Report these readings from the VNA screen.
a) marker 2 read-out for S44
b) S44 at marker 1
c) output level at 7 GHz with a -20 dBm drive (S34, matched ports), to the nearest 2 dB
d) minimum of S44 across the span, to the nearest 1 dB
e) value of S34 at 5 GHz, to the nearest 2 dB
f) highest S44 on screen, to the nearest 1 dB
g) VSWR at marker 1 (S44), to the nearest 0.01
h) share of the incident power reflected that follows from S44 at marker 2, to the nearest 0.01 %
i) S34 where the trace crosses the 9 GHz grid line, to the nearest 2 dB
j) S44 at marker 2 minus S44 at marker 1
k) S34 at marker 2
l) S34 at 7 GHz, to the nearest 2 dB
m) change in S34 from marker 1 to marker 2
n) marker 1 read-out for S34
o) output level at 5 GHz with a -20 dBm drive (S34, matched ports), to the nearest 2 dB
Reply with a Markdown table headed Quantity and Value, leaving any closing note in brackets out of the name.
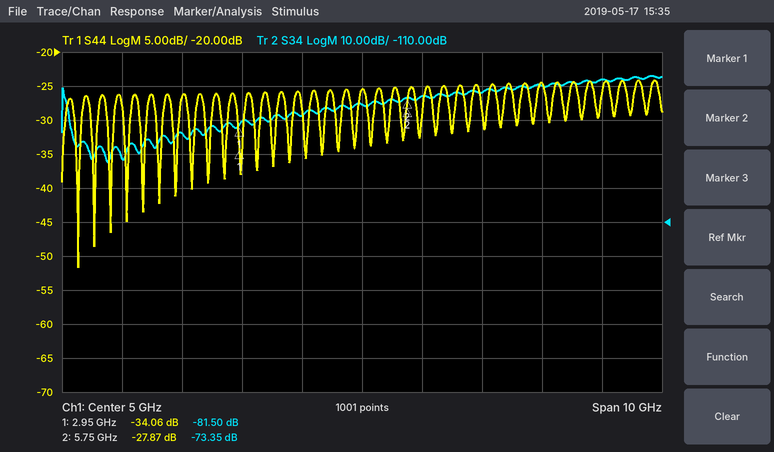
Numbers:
| Quantity | Value |
|---|---|
| marker 2 read-out for S44 | -27.87 dB |
| S44 at marker 1 | -34.06 dB |
| output level at 7 GHz with a -20 dBm drive (S34, matched ports), to the nearest 2 dB | -92 dBm |
| minimum of S44 across the span, to the nearest 1 dB | -52 dB |
| value of S34 at 5 GHz, to the nearest 2 dB | -76 dB |
| highest S44 on screen, to the nearest 1 dB | -24 dB |
| VSWR at marker 1 (S44), to the nearest 0.01 | 1.04 |
| share of the incident power reflected that follows from S44 at marker 2, to the nearest 0.01 % | 0.16 % |
| S34 where the trace crosses the 9 GHz grid line, to the nearest 2 dB | -68 dB |
| S44 at marker 2 minus S44 at marker 1 | 6.19 dB |
| S34 at marker 2 | -73.35 dB |
| S34 at 7 GHz, to the nearest 2 dB | -72 dB |
| change in S34 from marker 1 to marker 2 | 8.15 dB |
| marker 1 read-out for S34 | -81.50 dB |
| output level at 5 GHz with a -20 dBm drive (S34, matched ports), to the nearest 2 dB | -96 dBm |
